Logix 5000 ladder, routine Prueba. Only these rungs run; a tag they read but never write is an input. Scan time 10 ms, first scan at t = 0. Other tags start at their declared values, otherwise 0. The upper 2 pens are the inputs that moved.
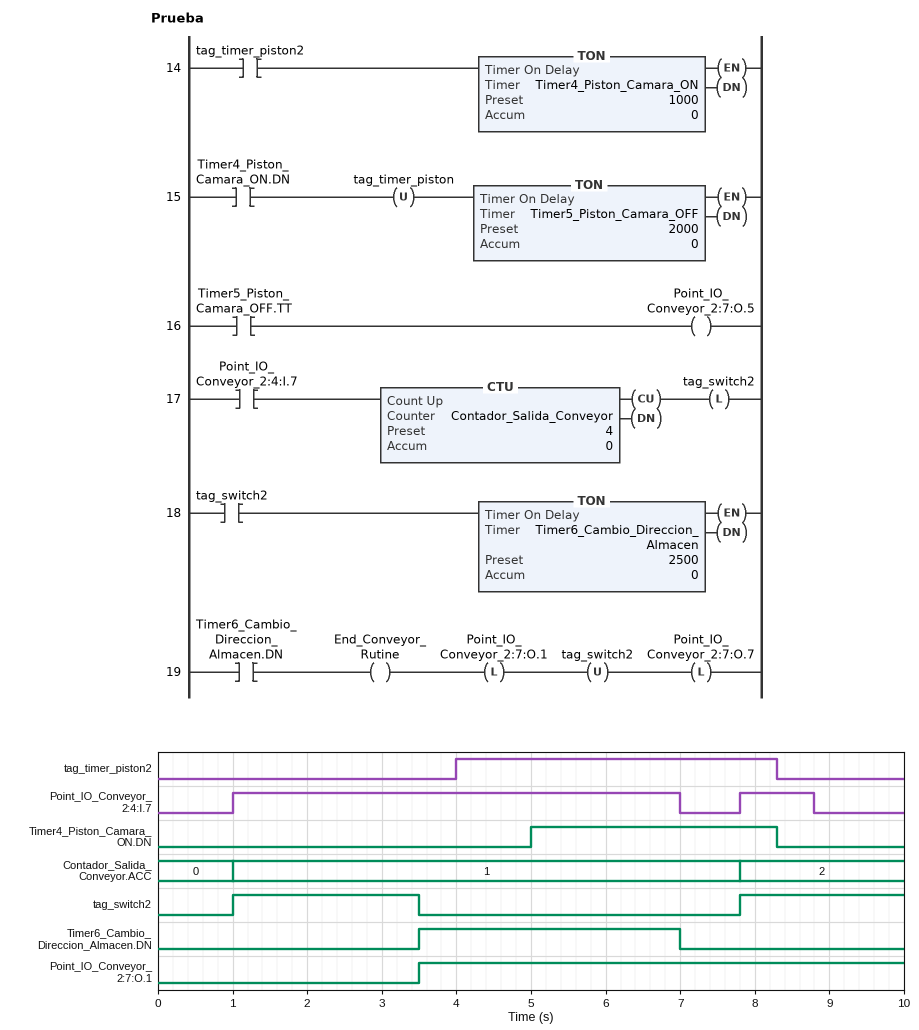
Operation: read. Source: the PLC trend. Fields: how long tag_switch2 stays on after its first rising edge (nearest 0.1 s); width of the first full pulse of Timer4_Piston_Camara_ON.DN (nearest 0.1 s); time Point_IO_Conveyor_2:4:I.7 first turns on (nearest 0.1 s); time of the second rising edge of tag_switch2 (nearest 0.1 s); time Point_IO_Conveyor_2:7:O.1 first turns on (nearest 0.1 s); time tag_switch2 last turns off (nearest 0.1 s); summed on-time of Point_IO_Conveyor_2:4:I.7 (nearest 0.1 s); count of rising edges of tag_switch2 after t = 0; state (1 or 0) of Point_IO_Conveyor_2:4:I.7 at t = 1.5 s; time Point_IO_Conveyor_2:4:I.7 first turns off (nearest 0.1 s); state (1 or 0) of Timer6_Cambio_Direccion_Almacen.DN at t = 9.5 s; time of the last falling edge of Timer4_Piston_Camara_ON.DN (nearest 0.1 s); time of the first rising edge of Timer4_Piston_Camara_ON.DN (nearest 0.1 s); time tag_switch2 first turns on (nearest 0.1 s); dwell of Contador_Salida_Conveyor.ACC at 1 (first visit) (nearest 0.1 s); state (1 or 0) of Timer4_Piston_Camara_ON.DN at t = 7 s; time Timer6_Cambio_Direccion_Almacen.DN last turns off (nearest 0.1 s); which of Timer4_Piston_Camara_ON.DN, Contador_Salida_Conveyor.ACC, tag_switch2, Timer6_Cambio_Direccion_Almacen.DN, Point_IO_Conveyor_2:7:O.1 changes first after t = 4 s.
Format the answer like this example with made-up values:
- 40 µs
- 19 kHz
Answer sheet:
- 2.5 s
- 3.3 s
- 1.0 s
- 7.8 s
- 3.5 s
- 3.5 s
- 7.0 s
- 2
- 1
- 7.0 s
- 0
- 8.3 s
- 5.0 s
- 1.0 s
- 6.8 s
- 1
- 7.0 s
- Timer4_Piston_Camara_ON.DN
